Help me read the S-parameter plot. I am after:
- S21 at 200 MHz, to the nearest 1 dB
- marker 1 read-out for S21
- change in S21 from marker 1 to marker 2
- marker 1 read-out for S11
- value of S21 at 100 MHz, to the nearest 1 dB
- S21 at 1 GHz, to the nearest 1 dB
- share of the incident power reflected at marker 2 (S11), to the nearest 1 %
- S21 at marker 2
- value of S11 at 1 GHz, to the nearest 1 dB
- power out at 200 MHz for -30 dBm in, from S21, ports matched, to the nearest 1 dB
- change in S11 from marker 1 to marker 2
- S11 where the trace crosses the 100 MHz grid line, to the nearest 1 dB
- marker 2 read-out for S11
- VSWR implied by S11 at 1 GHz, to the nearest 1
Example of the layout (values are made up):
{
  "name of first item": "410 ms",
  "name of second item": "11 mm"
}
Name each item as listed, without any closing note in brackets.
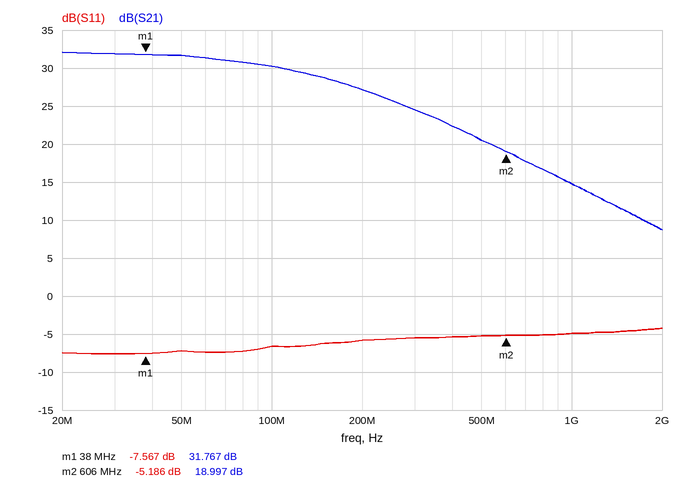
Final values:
{
  "S21 at 200 MHz, to the nearest 1 dB": "27 dB",
  "marker 1 read-out for S21": "31.767 dB",
  "change in S21 from marker 1 to marker 2": "-12.770 dB",
  "marker 1 read-out for S11": "-7.567 dB",
  "value of S21 at 100 MHz, to the nearest 1 dB": "30 dB",
  "S21 at 1 GHz, to the nearest 1 dB": "15 dB",
  "share of the incident power reflected at marker 2 (S11), to the nearest 1 %": "30 %",
  "S21 at marker 2": "18.997 dB",
  "value of S11 at 1 GHz, to the nearest 1 dB": "-5 dB",
  "power out at 200 MHz for -30 dBm in, from S21, ports matched, to the nearest 1 dB": "-3 dBm",
  "change in S11 from marker 1 to marker 2": "2.381 dB",
  "S11 where the trace crosses the 100 MHz grid line, to the nearest 1 dB": "-7 dB",
  "marker 2 read-out for S11": "-5.186 dB",
  "VSWR implied by S11 at 1 GHz, to the nearest 1": "4"
}
